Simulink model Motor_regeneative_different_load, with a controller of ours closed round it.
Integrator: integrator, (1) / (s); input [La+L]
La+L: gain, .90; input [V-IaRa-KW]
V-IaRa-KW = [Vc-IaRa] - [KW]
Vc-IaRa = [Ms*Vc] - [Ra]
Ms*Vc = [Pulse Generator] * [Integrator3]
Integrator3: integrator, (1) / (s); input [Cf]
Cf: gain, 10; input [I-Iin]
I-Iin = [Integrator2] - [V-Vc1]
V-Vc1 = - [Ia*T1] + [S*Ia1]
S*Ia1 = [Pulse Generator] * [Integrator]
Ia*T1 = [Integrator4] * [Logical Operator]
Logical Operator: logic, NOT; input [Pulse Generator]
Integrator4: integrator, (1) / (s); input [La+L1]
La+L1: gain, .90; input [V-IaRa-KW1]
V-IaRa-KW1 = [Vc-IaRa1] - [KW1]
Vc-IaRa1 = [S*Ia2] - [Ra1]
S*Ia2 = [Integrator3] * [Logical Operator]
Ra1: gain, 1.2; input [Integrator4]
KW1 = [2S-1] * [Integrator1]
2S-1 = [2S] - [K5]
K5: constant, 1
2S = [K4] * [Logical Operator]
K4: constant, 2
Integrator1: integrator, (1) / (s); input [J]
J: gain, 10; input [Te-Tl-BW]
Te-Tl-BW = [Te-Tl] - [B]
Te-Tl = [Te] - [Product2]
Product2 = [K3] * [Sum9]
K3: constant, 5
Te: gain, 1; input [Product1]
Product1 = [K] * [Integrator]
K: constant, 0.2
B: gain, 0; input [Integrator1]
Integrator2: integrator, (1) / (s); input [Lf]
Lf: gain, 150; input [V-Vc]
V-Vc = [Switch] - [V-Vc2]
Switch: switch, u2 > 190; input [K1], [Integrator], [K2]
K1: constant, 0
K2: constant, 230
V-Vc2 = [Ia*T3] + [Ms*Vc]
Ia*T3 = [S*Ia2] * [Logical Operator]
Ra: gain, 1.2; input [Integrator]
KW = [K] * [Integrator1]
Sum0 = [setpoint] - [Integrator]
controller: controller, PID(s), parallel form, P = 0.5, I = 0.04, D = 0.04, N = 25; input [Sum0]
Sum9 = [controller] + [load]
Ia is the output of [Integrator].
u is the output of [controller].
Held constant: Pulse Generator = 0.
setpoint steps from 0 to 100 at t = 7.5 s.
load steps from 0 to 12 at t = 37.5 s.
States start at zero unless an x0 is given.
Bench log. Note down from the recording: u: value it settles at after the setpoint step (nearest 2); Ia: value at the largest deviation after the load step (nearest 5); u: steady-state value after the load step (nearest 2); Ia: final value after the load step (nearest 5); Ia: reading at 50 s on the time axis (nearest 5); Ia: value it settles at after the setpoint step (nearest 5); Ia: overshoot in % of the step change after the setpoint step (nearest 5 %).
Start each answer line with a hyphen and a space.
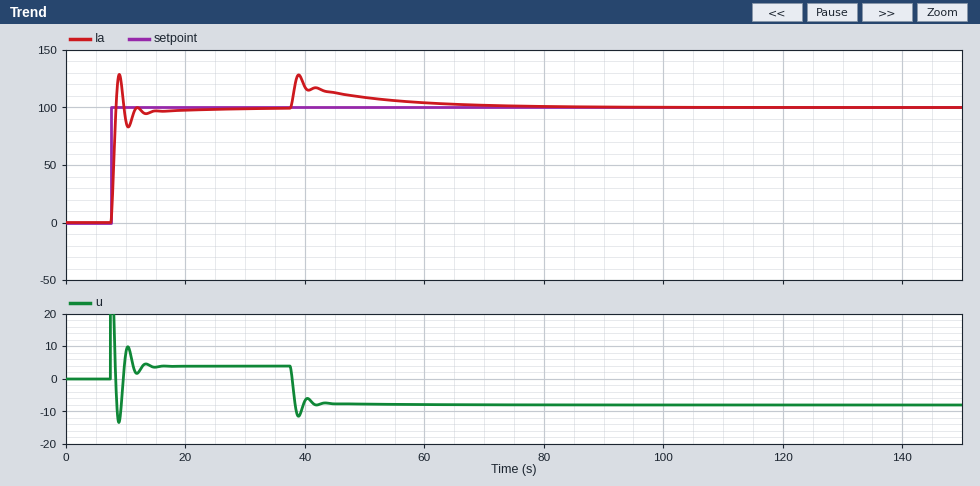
- 4
- 130
- -8
- 100
- 110
- 100
- 30 %
